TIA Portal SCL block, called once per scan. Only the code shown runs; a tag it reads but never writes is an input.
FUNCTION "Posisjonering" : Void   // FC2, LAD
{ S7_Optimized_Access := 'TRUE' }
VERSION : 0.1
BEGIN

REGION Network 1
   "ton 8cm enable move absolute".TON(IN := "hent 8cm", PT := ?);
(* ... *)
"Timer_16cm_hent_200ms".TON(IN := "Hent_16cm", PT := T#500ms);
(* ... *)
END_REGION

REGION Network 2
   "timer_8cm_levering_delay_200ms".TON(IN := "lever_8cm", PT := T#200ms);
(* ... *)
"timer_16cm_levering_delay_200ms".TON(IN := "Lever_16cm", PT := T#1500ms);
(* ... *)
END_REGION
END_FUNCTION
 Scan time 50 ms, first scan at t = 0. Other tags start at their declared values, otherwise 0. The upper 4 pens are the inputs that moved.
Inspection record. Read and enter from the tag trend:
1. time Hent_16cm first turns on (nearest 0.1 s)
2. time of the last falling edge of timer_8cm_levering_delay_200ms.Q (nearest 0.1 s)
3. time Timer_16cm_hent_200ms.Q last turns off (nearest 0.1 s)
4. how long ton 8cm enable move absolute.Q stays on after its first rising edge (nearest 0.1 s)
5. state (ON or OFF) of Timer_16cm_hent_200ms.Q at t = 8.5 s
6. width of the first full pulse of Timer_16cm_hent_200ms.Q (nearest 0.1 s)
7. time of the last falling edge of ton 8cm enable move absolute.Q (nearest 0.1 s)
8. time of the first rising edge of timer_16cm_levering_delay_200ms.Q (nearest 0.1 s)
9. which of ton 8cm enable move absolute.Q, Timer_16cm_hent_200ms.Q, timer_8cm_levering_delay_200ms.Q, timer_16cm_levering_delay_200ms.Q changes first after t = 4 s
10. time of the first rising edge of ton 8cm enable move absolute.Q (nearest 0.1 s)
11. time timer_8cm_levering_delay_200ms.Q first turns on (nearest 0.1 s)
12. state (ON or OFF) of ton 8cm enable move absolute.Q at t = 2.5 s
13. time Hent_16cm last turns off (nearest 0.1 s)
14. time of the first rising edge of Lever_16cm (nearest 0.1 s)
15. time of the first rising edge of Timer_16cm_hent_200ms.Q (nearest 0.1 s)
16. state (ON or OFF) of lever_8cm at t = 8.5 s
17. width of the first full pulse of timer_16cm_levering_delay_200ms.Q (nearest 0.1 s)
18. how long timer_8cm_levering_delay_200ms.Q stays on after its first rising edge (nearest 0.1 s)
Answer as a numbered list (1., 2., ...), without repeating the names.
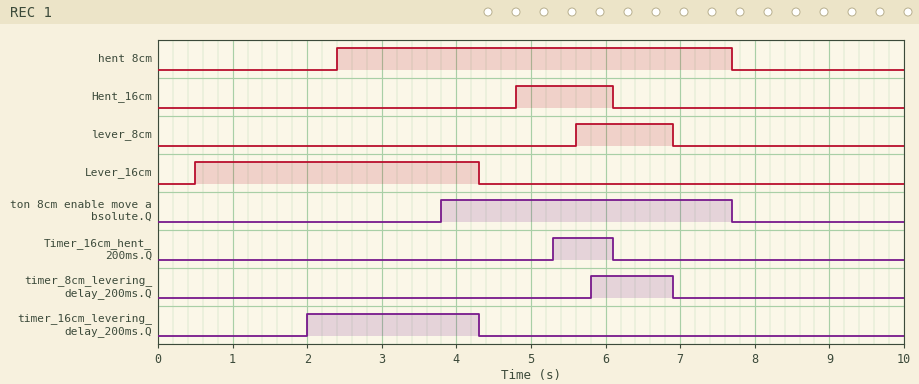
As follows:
1. 4.8 s
2. 6.9 s
3. 6.1 s
4. 3.9 s
5. OFF
6. 0.8 s
7. 7.7 s
8. 2.0 s
9. timer_16cm_levering_delay_200ms.Q
10. 3.8 s
11. 5.8 s
12. OFF
13. 6.1 s
14. 0.5 s
15. 5.3 s
16. OFF
17. 2.3 s
18. 1.1 s
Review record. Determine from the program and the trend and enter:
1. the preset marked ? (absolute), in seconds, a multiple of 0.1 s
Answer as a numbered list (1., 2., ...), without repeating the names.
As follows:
1. 1.4 s
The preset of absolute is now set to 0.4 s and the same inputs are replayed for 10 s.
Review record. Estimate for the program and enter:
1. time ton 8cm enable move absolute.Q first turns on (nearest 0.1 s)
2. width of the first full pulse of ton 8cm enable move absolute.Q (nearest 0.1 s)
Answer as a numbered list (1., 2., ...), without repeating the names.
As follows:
1. 2.8 s
2. 4.9 s
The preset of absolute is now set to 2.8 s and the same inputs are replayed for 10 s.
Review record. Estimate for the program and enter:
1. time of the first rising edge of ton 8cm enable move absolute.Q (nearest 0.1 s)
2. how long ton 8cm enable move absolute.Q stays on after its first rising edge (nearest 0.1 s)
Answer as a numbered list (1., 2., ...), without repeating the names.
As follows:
1. 5.2 s
2. 2.5 s
